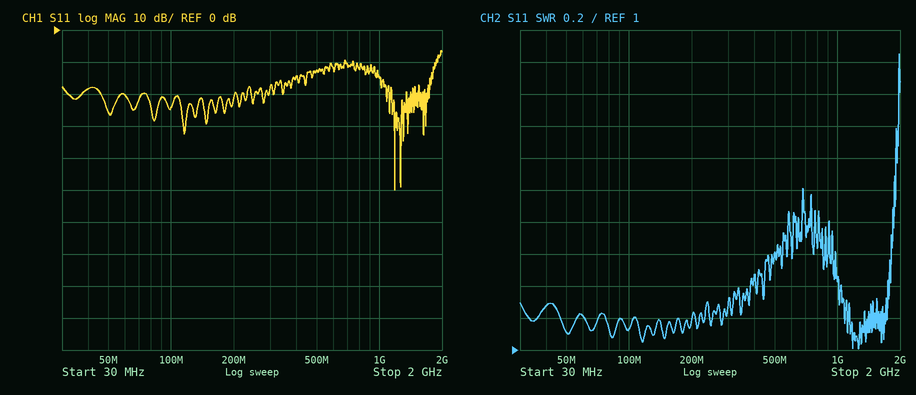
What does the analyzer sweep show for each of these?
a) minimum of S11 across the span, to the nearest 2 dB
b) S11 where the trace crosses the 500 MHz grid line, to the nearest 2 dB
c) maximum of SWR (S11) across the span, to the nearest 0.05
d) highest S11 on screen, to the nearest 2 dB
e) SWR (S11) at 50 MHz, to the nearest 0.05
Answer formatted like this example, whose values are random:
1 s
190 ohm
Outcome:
-50 dB
-12 dB
2.85
-6 dB
1.10
